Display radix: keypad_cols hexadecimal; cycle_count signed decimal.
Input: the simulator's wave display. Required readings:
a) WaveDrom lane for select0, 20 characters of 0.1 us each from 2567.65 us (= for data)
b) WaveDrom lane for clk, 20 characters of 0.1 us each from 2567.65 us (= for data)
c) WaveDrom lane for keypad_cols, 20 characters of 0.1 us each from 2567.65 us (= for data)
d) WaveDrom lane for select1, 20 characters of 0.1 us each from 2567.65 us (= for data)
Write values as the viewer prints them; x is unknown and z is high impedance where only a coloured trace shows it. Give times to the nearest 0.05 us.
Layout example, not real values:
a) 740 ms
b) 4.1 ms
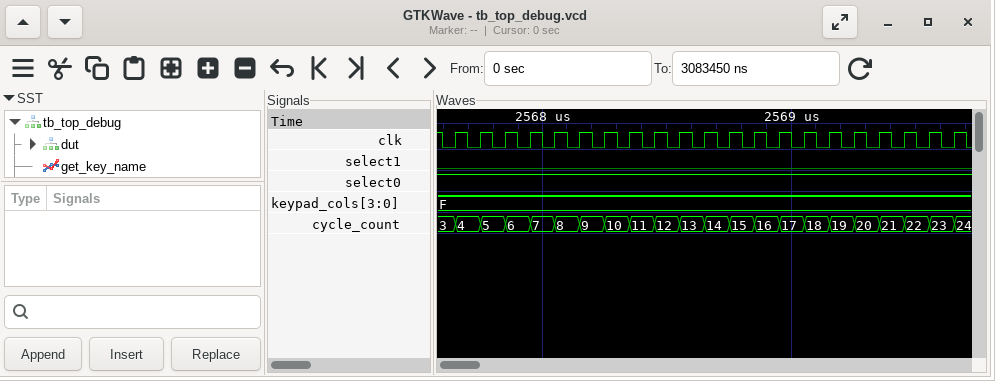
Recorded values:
a) {name: 'select0', wave: '1...................'}
b) {name: 'clk', wave: 'p...................'}
c) {name: 'keypad_cols', wave: '=...................', data: 'F'}
d) {name: 'select1', wave: '0...................'}
